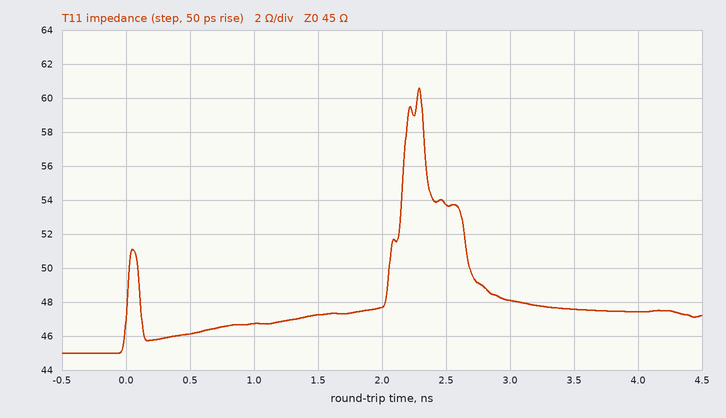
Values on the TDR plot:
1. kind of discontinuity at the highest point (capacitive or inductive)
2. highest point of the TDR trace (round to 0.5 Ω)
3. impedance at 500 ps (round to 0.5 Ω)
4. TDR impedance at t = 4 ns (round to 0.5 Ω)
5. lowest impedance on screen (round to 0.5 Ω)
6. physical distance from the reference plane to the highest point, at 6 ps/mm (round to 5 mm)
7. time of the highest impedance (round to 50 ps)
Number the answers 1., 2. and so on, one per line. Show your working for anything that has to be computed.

1. inductive
2. 60.5 Ω
3. 46.0 Ω
4. 47.5 Ω
5. 45.0 Ω
6. 2.30 ns / 2 / 6 ps/mm ≈ 192 mm, so 190 mm to the nearest 5 mm
7. 2.30 ns
